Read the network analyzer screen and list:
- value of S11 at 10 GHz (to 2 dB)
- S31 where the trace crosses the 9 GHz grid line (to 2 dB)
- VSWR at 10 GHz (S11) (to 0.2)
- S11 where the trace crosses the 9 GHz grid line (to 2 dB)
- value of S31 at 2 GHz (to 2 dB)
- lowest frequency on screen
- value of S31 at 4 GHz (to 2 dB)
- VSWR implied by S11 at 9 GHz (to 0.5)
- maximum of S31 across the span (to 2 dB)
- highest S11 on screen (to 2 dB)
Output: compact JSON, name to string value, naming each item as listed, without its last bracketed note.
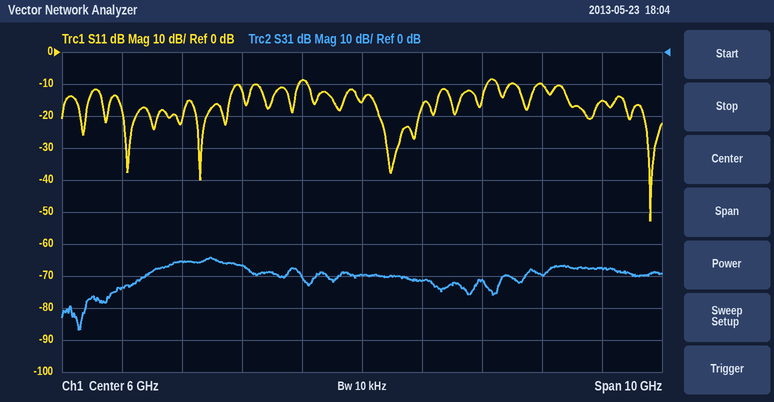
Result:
{"value of S11 at 10 GHz": "-16 dB", "S31 where the trace crosses the 9 GHz grid line": "-70 dB", "VSWR at 10 GHz (S11)": "1.4", "S11 where the trace crosses the 9 GHz grid line": "-10 dB", "value of S31 at 2 GHz": "-74 dB", "lowest frequency on screen": "1 GHz", "value of S31 at 4 GHz": "-66 dB", "VSWR implied by S11 at 9 GHz": "2.0", "maximum of S31 across the span": "-64 dB", "highest S11 on screen": "-8 dB"}
